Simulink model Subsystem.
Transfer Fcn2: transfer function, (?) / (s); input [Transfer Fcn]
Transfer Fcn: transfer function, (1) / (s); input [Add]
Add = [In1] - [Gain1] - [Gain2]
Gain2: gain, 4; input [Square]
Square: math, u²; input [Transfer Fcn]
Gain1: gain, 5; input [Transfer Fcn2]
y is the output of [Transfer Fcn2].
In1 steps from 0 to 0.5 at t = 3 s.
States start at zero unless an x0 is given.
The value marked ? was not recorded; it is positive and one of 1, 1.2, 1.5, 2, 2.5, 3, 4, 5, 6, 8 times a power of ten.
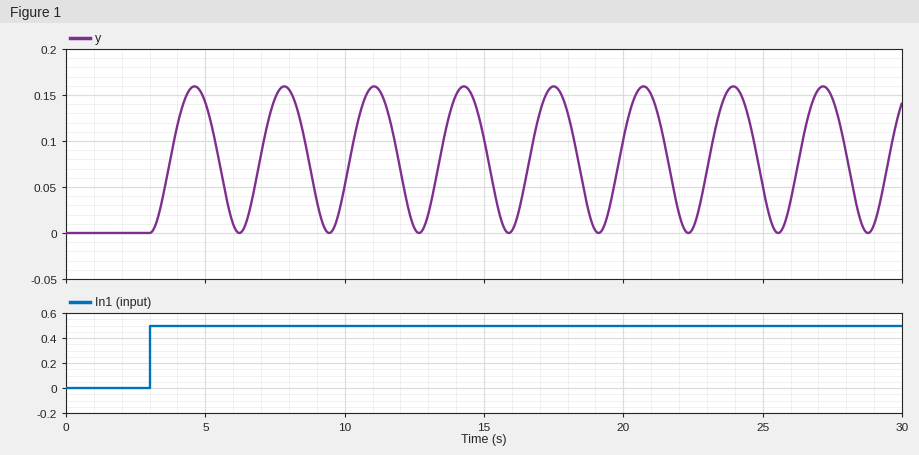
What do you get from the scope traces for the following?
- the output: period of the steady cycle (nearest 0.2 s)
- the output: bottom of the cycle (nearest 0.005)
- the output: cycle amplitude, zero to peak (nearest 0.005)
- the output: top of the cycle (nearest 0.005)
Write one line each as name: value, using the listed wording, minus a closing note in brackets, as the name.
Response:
the output: period of the steady cycle: 3.2 s
the output: bottom of the cycle: 0.000
the output: cycle amplitude, zero to peak: 0.080
the output: top of the cycle: 0.160
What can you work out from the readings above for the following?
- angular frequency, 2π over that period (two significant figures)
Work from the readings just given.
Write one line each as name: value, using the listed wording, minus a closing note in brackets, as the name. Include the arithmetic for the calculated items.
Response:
angular frequency, 2π over that period: 2π / 3.2 = 2.0 rad/s
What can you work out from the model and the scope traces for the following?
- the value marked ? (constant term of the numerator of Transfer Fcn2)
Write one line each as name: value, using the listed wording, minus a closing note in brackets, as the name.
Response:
the value marked ?: 0.8
